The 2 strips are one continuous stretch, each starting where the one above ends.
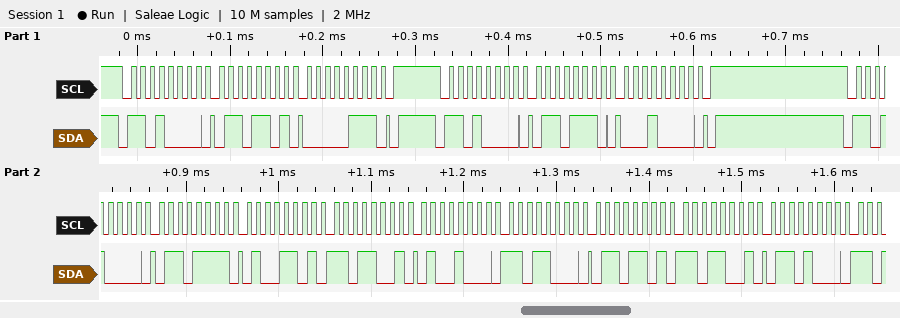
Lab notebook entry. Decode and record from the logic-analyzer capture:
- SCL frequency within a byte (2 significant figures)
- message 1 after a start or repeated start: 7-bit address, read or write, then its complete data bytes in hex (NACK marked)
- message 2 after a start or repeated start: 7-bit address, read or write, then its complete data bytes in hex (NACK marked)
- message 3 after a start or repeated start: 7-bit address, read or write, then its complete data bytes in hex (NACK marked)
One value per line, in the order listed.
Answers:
100 kHz
0x68 write: 6D 07
0x68 write: 6E 10
0x68 write: 6F 4D D9 48 D8 6D D9 68
